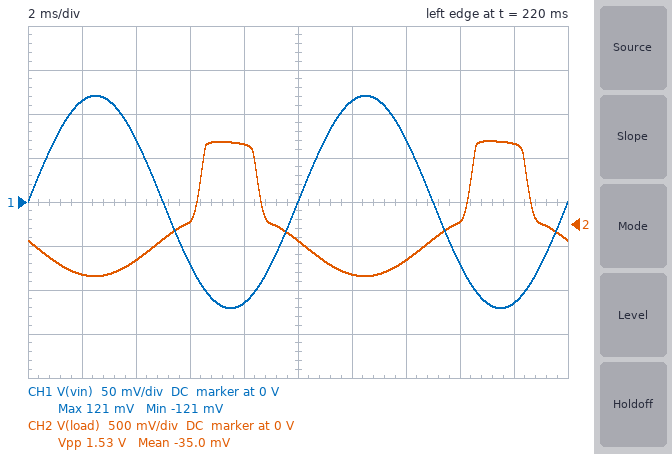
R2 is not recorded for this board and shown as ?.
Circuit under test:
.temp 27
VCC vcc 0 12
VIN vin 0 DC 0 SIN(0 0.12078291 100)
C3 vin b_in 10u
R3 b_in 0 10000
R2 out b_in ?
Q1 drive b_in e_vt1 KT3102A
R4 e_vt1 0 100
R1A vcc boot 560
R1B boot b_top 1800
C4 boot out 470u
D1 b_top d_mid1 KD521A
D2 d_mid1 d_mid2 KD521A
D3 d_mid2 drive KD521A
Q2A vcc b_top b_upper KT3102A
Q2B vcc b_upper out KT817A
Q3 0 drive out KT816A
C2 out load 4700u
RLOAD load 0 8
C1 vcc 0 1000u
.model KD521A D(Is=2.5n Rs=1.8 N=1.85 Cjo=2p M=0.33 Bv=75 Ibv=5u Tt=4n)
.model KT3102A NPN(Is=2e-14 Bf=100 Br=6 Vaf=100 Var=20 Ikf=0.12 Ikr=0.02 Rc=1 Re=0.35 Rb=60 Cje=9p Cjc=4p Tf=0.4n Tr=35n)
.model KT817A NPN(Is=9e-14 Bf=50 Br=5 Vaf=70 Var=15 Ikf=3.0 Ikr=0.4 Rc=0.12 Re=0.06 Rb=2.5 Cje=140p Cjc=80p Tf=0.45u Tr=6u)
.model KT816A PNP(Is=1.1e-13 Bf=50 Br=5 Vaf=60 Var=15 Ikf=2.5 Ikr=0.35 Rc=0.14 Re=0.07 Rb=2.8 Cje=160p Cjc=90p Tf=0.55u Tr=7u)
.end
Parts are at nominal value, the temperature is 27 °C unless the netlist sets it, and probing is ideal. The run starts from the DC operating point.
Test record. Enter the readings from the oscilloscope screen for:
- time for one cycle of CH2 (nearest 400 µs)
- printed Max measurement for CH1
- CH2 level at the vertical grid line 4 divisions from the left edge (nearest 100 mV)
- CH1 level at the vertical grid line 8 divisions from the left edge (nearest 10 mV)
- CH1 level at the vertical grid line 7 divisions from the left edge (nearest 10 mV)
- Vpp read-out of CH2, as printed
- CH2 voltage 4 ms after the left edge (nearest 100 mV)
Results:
10.0 ms
121 mV
900 mV
-70 mV
70 mV
1.53 V
-400 mV
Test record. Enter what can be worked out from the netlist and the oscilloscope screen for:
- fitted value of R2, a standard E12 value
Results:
120 kΩ
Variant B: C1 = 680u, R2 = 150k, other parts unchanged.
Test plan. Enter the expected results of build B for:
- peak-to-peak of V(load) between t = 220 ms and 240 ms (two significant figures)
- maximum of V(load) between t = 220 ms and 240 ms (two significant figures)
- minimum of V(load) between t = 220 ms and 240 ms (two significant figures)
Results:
690 mV
300 mV
-380 mV
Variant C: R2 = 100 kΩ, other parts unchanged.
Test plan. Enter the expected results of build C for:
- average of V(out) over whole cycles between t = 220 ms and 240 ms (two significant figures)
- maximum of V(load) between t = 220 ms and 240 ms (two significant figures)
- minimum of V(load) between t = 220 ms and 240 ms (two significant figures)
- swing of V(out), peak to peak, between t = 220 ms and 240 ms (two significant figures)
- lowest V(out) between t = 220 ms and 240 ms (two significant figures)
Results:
9.6 V
1.5 V
-690 mV
2.2 V
9.0 V
